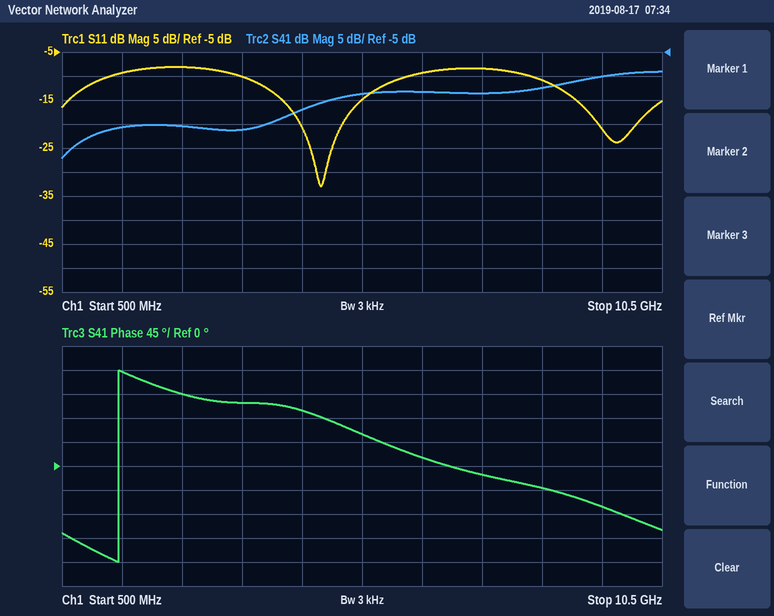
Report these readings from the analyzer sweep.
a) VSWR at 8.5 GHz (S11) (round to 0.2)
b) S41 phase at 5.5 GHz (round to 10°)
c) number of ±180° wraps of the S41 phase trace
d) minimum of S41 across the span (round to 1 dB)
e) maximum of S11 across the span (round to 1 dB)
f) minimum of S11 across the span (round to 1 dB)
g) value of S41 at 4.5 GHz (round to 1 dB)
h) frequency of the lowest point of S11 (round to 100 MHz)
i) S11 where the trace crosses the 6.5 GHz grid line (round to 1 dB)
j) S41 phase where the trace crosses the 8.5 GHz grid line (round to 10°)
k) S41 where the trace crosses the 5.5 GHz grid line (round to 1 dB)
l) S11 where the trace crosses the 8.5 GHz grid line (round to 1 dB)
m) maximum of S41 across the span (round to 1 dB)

1.8
60°
1
-27 dB
-8 dB
-33 dB
-17 dB
4.8 GHz
-9 dB
-40°
-14 dB
-11 dB
-9 dB
